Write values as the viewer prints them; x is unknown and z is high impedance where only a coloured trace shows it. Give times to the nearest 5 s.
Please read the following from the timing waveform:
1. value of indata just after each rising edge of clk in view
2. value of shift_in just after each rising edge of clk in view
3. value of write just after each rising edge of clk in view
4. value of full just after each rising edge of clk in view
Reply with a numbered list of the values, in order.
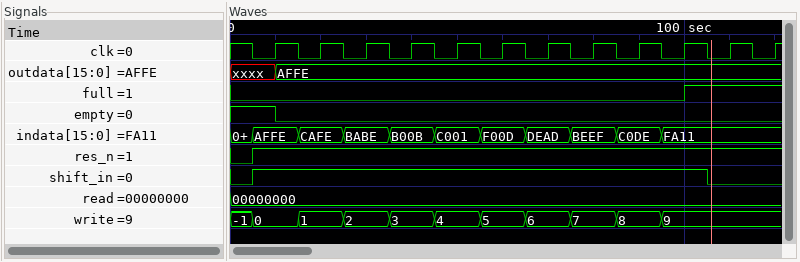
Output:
1. AFFE, CAFE, BABE, B00B, C001, F00D, DEAD, BEEF, C0DE, FA11, FA11, FA11
2. 1 1 1 1 1 1 1 1 1 1 0 0
3. 0, 1, 2, 3, 4, 5, 6, 7, 8, 9, 9, 9
4. 0 0 0 0 0 0 0 0 0 1 1 1
